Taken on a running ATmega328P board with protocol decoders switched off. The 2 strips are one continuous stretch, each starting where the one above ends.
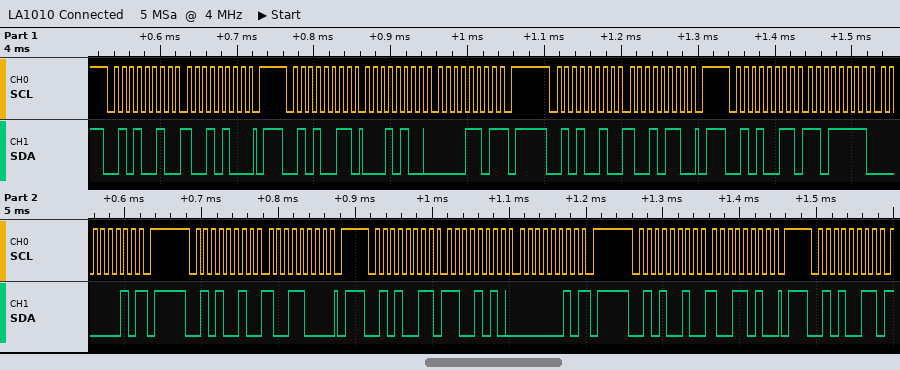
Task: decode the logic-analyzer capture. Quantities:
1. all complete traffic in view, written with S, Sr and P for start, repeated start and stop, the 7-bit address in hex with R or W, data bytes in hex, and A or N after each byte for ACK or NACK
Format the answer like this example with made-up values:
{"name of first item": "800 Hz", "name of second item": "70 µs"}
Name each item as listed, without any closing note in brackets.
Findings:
{"all complete traffic in view, written with S, Sr and P for start, repeated start and stop, the 7-bit address in hex with R or W, data bytes in hex, and A or N after each byte for ACK or NACK": "S 29W A 94 A P S 29R A 14 A 0D N P S 29W A 96 A P S 29R A DF A 02 N P S 29W A 98 A P S 29R A CA A 02 N P S 29W A 9A A P S 29R A"}
